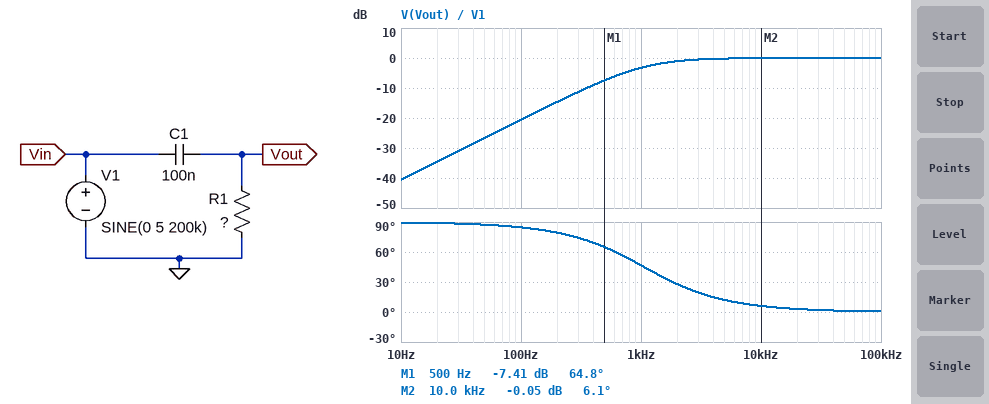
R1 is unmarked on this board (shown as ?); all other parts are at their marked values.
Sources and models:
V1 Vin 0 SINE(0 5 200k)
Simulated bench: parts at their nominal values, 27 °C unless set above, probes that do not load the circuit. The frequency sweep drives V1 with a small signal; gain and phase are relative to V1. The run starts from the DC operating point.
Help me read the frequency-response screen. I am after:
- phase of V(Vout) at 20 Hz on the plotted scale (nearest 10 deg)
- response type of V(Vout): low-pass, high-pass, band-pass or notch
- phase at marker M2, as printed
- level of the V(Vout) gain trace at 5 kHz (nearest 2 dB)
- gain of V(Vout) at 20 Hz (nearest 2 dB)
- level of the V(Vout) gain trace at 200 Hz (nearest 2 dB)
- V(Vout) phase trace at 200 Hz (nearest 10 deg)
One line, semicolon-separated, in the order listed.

90 deg; high-pass; 6.1 deg; 0 dB; -34 dB; -14 dB; 80 deg
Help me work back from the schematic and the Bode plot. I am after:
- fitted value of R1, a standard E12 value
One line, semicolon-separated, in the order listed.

1.5 kΩ
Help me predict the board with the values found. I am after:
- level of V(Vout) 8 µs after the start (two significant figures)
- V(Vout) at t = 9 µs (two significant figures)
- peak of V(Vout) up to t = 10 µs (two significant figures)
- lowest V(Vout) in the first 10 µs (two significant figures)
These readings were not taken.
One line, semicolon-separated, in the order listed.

-3.0 V; -4.8 V; 5.0 V; -5.0 V
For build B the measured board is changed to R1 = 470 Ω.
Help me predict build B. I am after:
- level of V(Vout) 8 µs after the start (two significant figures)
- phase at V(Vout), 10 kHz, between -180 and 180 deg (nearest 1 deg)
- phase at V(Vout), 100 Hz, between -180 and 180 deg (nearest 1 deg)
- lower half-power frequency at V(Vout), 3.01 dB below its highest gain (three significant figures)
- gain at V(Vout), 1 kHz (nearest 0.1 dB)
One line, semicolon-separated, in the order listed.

-3.1 V; 19 deg; 88 deg; 3.39 kHz; -11.0 dB
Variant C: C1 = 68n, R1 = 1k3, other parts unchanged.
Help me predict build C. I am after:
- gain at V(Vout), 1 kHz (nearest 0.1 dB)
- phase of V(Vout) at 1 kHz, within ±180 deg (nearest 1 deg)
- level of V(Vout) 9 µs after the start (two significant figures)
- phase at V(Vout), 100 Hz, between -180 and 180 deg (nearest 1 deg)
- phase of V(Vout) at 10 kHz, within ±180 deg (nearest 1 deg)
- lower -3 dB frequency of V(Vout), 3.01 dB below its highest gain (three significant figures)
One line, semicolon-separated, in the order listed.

-6.3 dB; 61 deg; -4.8 V; 87 deg; 10 deg; 1.80 kHz
